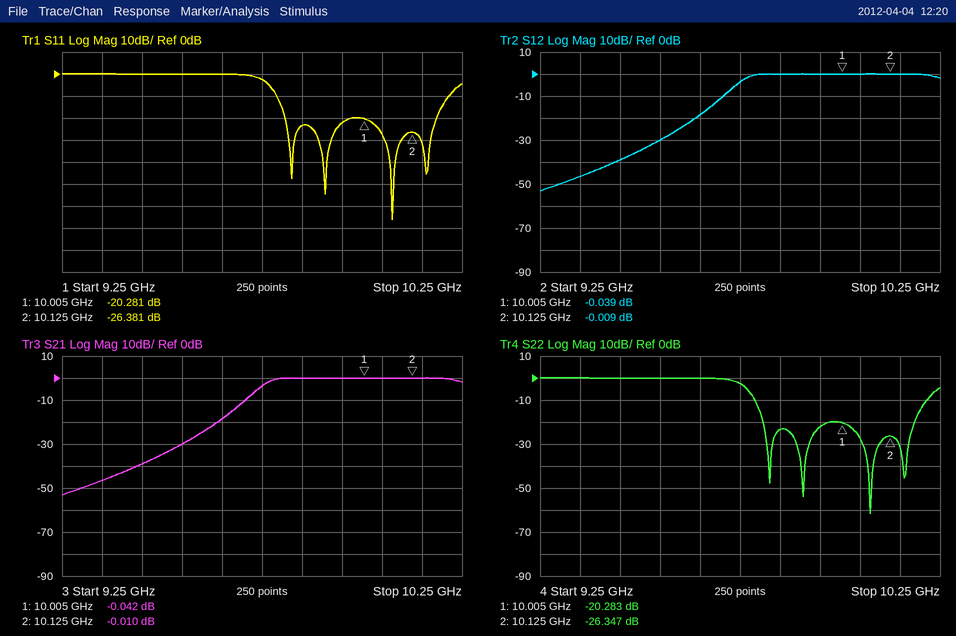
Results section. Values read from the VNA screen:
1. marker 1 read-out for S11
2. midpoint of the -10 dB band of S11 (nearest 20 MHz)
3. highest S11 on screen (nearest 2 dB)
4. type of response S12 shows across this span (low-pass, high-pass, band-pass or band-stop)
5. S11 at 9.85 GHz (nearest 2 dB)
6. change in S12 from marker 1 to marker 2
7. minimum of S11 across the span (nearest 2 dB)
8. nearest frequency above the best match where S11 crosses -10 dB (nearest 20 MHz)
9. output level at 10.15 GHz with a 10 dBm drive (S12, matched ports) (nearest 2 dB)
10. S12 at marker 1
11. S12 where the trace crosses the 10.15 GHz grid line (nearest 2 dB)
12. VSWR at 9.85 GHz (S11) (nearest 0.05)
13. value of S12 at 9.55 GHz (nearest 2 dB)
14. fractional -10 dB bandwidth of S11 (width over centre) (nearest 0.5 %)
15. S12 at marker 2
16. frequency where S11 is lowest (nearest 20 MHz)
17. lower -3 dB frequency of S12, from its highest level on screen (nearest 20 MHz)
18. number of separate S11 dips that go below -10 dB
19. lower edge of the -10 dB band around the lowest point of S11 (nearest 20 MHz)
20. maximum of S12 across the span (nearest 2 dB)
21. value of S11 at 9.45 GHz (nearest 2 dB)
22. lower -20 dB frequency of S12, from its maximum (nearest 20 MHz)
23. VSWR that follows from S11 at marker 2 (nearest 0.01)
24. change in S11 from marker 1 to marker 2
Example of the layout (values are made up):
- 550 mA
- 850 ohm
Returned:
- -20.281 dB
- 10.00 GHz
- 0 dB
- high-pass
- -24 dB
- 0.030 dB
- -66 dB
- 10.22 GHz
- 10 dBm
- -0.039 dB
- 0 dB
- 1.15
- -30 dB
- 4.5 %
- -0.009 dB
- 10.08 GHz
- 9.76 GHz
- 4
- 9.78 GHz
- 0 dB
- 0 dB
- 9.64 GHz
- 1.10
- -6.100 dB
